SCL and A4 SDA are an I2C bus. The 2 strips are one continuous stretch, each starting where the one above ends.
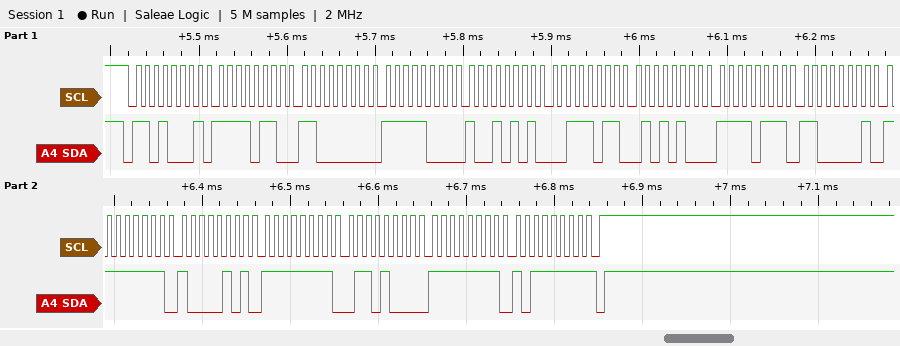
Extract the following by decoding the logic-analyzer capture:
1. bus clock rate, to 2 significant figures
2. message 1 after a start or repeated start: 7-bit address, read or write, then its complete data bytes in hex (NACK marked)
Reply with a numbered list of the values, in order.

1. 100 kHz
2. 0x68 read: F6 C0 F8 95 3B 54 F7 C1 FF 85 FF 68 FF BF NACK
